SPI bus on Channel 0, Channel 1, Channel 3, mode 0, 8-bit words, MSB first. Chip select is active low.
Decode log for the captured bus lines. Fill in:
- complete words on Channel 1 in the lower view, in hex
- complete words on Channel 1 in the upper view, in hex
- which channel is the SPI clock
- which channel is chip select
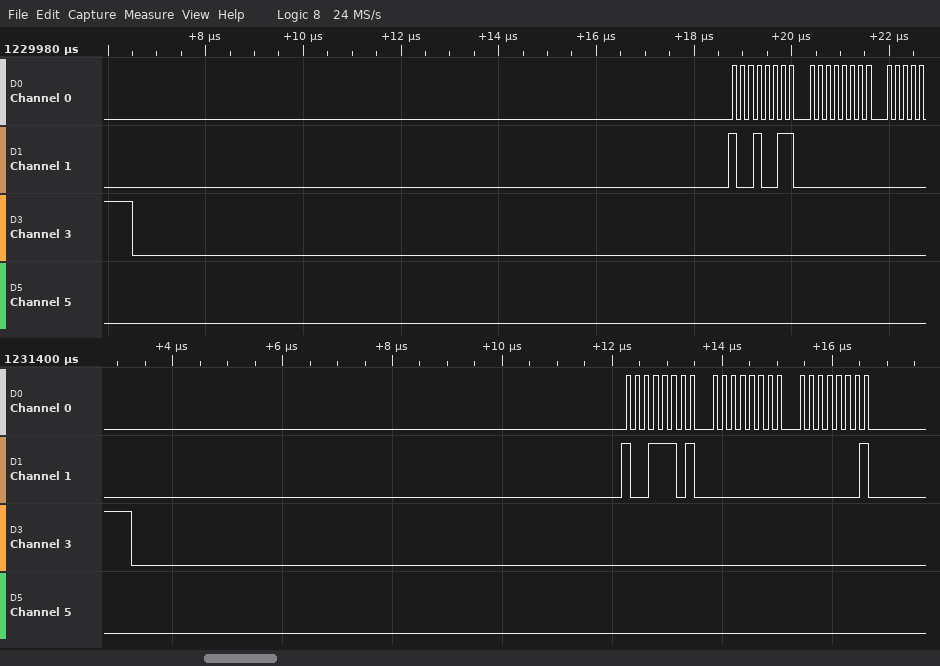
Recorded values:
9D, 00, 01
93, 00
Channel 0
Channel 3
